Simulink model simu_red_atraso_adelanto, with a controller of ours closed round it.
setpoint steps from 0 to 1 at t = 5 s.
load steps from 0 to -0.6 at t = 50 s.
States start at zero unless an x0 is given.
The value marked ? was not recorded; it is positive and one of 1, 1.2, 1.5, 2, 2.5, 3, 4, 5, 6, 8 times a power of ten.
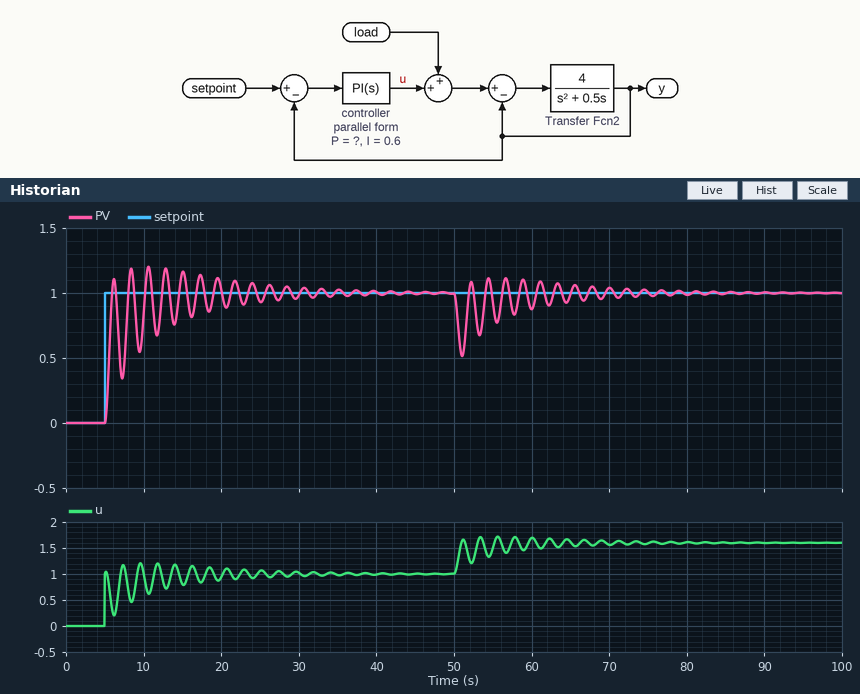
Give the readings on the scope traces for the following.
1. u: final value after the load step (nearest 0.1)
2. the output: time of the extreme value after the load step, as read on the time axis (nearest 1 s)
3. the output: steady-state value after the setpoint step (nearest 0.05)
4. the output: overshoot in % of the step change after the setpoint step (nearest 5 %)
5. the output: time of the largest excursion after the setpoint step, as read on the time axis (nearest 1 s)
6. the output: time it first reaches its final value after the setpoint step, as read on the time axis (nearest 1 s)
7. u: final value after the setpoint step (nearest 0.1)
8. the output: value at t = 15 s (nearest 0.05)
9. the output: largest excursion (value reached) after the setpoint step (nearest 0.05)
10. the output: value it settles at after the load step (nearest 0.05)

1.6
51 s
1.00
20 %
11 s
6 s
1.0
1.15
1.20
1.00
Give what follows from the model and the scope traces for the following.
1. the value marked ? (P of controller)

1
